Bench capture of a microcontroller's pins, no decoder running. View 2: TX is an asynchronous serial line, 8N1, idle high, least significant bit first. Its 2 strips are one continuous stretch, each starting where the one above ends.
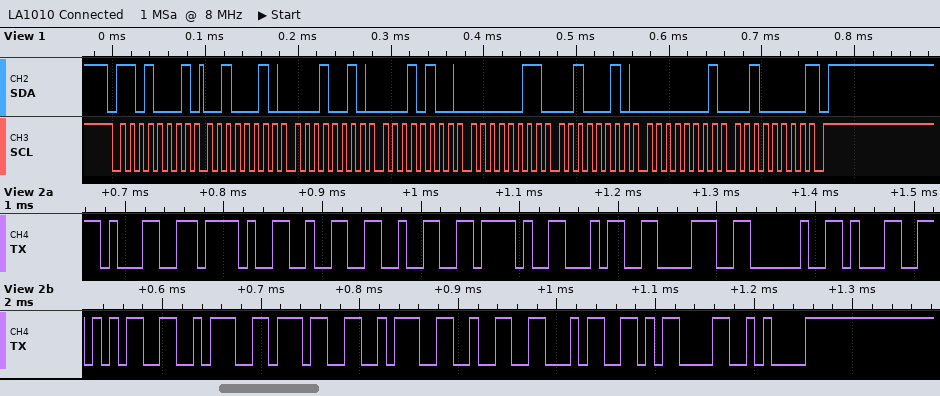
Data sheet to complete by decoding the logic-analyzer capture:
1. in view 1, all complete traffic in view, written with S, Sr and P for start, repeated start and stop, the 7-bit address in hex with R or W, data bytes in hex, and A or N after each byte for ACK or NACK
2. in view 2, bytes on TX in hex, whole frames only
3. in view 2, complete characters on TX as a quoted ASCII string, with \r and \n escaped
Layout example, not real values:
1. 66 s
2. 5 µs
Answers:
1. S 68R A 22 A 12 A 14 A 03 A 22 A 01 A 20 N P
2. 0x31 0x2F 0x32 0x32 0x2F 0x34 0x38 0x20 0x31 0x35 0x3A 0x37 0x3A 0x32 0x34 0x0D 0x0A
3. "1/22/48 15:7:24\r\n"
